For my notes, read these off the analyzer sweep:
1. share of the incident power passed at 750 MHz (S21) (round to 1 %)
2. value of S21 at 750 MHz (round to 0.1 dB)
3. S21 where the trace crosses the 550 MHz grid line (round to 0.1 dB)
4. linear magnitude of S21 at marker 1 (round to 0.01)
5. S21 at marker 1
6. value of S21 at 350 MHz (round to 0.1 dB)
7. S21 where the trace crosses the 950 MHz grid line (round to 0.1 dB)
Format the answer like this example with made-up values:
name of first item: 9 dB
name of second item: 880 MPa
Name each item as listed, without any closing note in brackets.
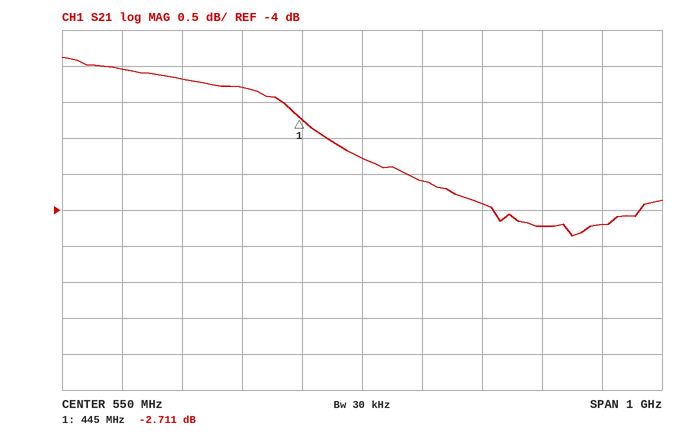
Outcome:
share of the incident power passed at 750 MHz (S21): 41 %
value of S21 at 750 MHz: -3.9 dB
S21 where the trace crosses the 550 MHz grid line: -3.3 dB
linear magnitude of S21 at marker 1: 0.73
S21 at marker 1: -2.711 dB
value of S21 at 350 MHz: -2.3 dB
S21 where the trace crosses the 950 MHz grid line: -4.2 dB
